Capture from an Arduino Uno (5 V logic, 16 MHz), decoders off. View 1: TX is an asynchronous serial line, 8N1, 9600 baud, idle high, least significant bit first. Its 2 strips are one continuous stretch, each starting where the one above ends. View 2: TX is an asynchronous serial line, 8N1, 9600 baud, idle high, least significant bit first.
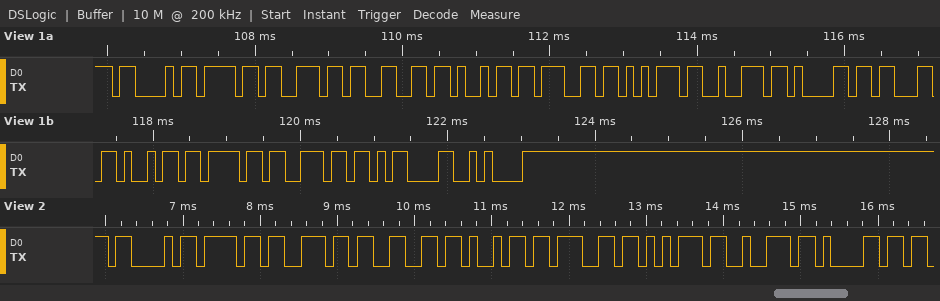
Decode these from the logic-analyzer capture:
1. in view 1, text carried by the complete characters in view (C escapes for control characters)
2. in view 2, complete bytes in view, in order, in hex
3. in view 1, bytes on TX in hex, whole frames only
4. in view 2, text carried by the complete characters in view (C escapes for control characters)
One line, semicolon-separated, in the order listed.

"Configuracion\r\n"; 0x43 0x6F 0x6E 0x66 0x69 0x67 0x75 0x72 0x61; 0x43 0x6F 0x6E 0x66 0x69 0x67 0x75 0x72 0x61 0x63 0x69 0x6F 0x6E 0x0D 0x0A; "Configura"
